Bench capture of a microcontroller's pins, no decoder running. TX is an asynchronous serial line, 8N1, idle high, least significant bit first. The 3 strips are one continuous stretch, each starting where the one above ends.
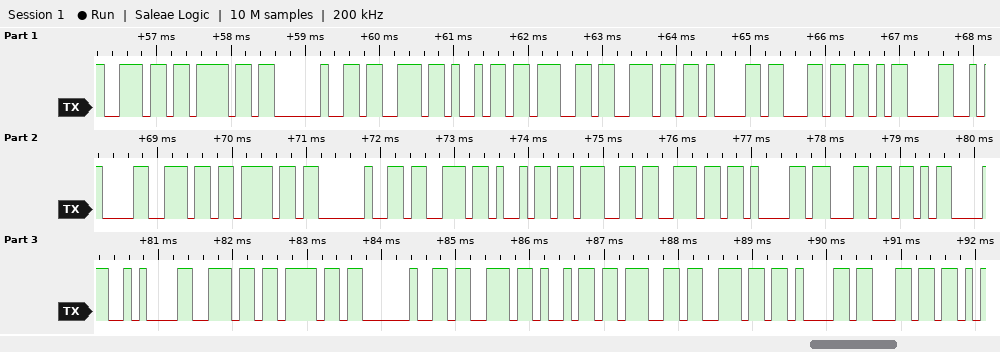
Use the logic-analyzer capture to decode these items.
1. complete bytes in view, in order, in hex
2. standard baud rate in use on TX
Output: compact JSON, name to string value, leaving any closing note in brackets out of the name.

{"complete bytes in view, in order, in hex": "6E 6F 20 73 69 67 6E 61 6C 0D 0A 6E 6F 20 73 69 67 6E 61 6C 0D 0A 6E 6F 20 73 69 67 6E 61 6C", "standard baud rate in use on TX": "9600 baud"}
